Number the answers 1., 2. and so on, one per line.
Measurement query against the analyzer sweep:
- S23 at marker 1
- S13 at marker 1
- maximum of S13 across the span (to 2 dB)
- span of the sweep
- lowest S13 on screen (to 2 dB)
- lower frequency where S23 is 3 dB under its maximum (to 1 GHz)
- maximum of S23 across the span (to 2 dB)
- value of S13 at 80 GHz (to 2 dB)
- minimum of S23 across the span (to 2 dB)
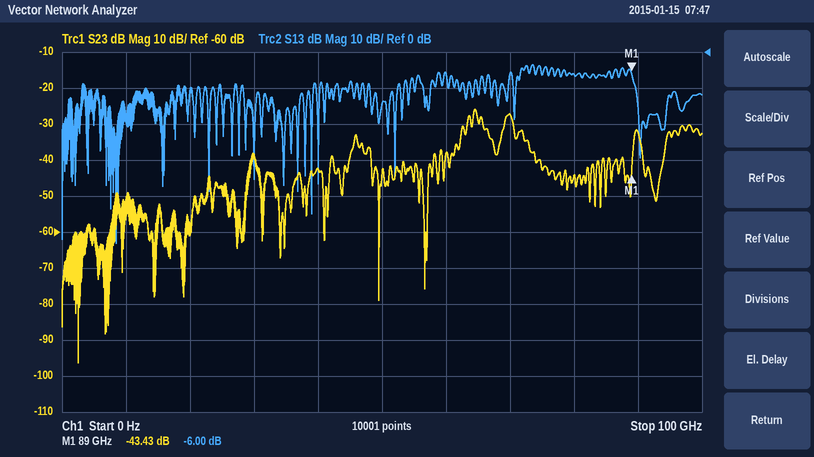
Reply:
1. -43.43 dB
2. -6.00 dB
3. -4 dB
4. 100 GHz
5. -54 dB
6. 64 GHz
7. -26 dB
8. -6 dB
9. -96 dB
